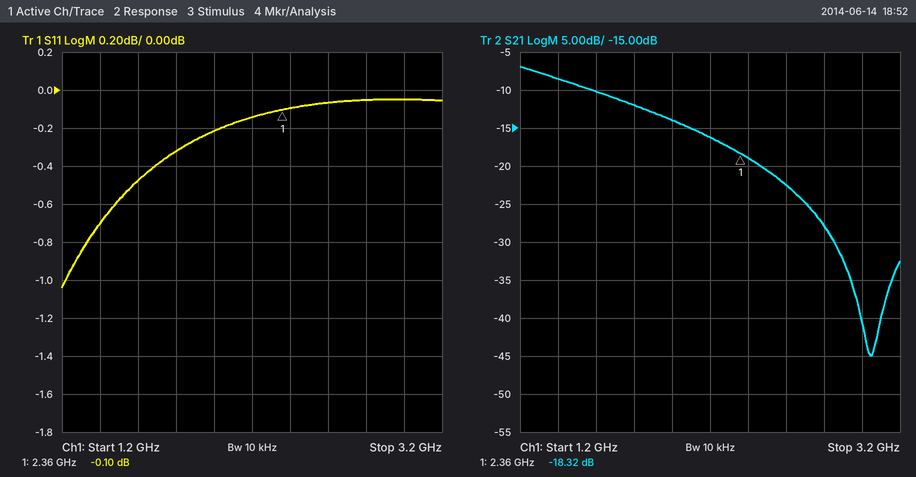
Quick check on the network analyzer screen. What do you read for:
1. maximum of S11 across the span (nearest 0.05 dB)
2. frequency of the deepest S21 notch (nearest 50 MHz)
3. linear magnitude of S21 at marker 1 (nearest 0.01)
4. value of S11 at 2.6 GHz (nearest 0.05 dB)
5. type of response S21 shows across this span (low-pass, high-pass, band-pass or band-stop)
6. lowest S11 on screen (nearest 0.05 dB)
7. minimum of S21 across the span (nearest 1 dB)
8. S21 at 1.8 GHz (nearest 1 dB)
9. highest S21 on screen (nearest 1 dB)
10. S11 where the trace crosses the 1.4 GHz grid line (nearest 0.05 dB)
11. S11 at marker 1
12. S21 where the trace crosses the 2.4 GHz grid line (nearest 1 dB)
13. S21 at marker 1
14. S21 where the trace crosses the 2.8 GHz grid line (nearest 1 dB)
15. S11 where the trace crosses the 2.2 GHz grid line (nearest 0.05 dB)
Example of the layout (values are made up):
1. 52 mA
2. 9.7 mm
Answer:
1. -0.05 dB
2. 3.05 GHz
3. 0.12
4. -0.05 dB
5. low-pass
6. -1.05 dB
7. -45 dB
8. -12 dB
9. -7 dB
10. -0.70 dB
11. -0.10 dB
12. -19 dB
13. -18.32 dB
14. -28 dB
15. -0.15 dB
